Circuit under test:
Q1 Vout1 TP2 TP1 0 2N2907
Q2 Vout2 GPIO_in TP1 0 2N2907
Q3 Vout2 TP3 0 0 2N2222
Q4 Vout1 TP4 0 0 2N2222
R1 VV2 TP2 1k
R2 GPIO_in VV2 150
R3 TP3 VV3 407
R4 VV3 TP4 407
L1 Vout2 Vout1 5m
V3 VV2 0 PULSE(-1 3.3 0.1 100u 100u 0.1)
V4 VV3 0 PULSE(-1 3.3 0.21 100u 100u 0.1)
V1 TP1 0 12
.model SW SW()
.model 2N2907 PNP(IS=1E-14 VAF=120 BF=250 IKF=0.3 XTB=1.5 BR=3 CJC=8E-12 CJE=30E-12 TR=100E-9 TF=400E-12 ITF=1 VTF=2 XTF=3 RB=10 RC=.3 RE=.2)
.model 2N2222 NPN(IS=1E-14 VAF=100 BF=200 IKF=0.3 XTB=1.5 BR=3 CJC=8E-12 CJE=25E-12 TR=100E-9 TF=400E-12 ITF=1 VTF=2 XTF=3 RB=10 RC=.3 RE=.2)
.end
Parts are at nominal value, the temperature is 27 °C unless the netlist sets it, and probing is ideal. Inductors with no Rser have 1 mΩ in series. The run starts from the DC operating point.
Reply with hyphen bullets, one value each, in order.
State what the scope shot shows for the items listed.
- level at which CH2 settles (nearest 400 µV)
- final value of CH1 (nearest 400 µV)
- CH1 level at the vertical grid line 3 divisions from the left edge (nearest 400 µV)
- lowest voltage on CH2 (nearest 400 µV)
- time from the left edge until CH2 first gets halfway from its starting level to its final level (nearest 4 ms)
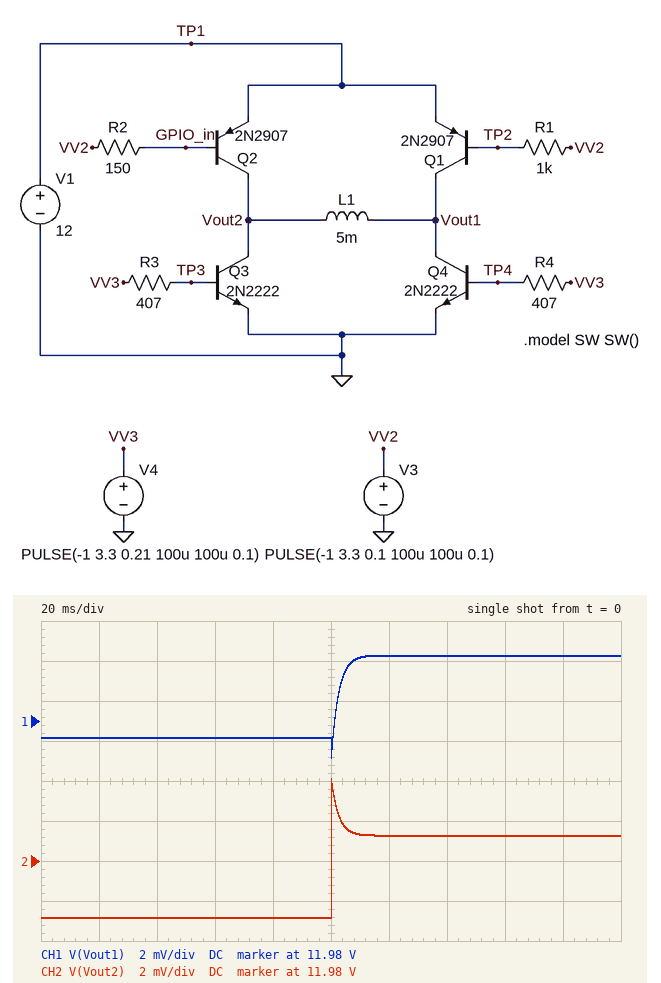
- 11.9832 V
- 11.9832 V
- 11.9792 V
- 11.9792 V
- 100 ms
